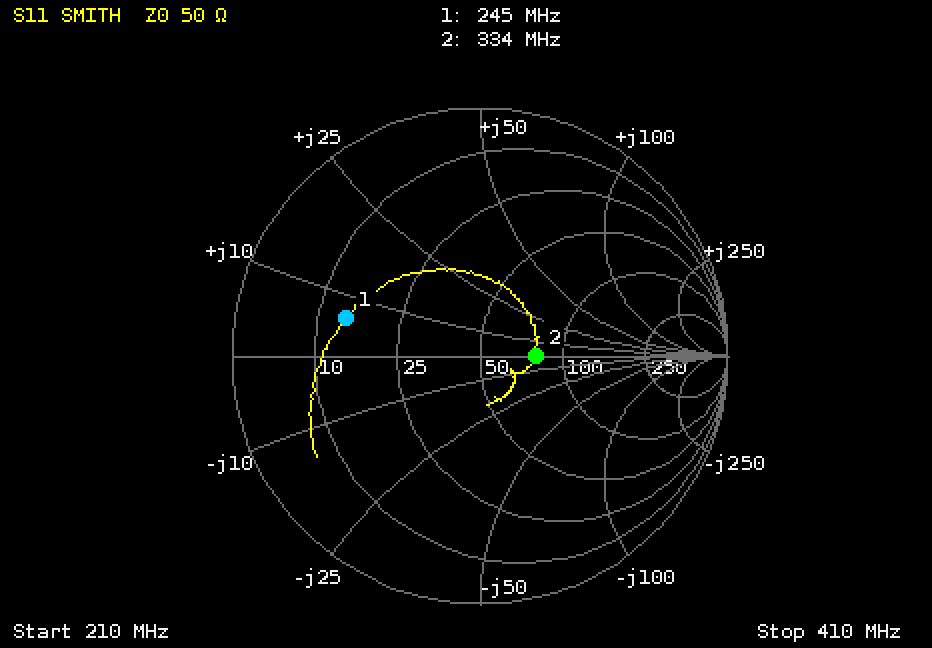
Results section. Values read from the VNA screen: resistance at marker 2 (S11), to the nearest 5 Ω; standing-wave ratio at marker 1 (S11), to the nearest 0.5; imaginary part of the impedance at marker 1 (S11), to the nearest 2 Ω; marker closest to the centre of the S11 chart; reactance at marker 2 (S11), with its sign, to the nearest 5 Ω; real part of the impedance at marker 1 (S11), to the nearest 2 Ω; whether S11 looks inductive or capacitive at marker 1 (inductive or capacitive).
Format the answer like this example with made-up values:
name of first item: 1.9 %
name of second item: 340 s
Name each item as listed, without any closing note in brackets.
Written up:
resistance at marker 2 (S11), to the nearest 5 Ω: 80 Ω
standing-wave ratio at marker 1 (S11), to the nearest 0.5: 3.5
imaginary part of the impedance at marker 1 (S11), to the nearest 2 Ω: +6 Ω
marker closest to the centre of the S11 chart: marker 2
reactance at marker 2 (S11), with its sign, to the nearest 5 Ω: 0 Ω
real part of the impedance at marker 1 (S11), to the nearest 2 Ω: 14 Ω
whether S11 looks inductive or capacitive at marker 1: inductive
